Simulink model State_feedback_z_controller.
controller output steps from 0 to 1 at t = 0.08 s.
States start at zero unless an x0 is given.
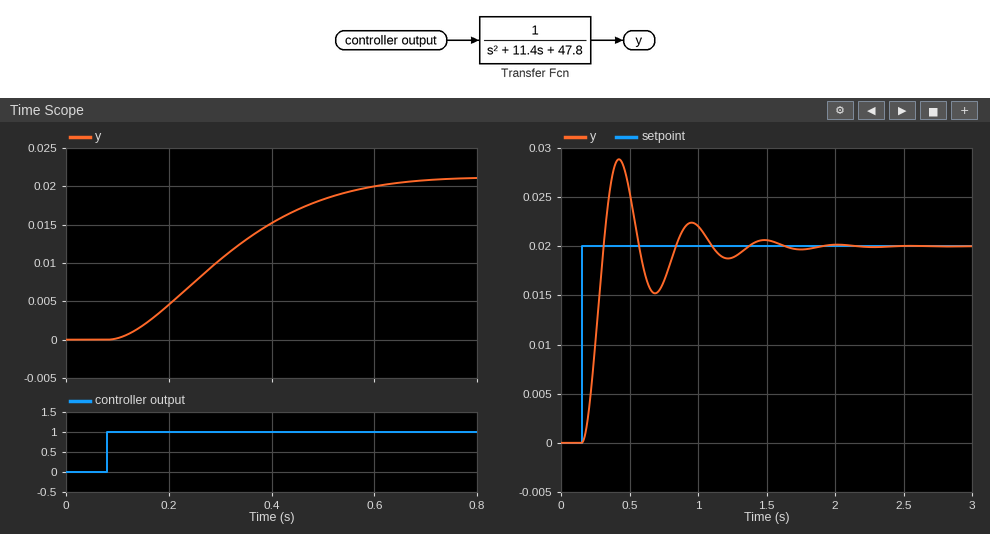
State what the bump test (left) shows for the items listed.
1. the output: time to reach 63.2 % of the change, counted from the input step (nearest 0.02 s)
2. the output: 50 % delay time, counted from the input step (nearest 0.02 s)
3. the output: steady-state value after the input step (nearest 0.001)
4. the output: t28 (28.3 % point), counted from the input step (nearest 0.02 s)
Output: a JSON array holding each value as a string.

["0.28 s", "0.22 s", "0.021", "0.14 s"]
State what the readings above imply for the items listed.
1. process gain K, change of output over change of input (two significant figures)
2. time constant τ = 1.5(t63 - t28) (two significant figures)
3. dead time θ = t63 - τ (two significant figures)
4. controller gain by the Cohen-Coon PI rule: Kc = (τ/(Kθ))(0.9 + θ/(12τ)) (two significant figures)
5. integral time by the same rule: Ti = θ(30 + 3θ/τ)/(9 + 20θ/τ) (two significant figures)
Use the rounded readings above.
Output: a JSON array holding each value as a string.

["0.021", "0.21 s", "0.070 s", "130", "0.14 s"]
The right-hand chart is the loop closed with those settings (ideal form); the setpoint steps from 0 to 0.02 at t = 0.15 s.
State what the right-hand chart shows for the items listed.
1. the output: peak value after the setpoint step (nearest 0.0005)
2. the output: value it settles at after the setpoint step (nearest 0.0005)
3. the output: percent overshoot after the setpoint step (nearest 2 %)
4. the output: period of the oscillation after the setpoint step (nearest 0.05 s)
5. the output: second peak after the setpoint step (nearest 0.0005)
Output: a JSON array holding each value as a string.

["0.0290", "0.0200", "44 %", "0.55 s", "0.0225"]
